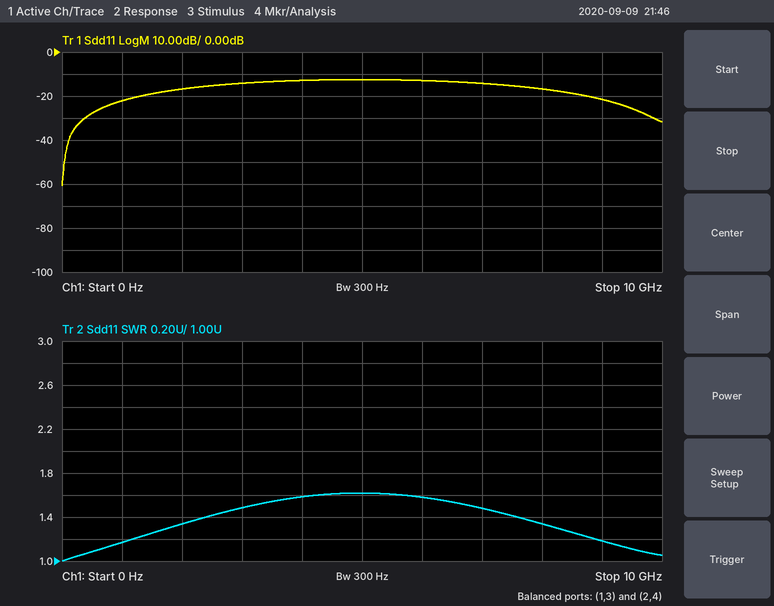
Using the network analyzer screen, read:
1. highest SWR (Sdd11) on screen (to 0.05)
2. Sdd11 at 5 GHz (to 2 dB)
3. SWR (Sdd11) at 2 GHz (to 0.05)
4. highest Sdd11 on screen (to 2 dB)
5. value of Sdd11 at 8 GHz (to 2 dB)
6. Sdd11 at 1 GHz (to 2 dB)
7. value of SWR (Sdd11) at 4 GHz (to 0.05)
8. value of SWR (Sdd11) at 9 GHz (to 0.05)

1.60
-12 dB
1.35
-12 dB
-16 dB
-22 dB
1.60
1.20
